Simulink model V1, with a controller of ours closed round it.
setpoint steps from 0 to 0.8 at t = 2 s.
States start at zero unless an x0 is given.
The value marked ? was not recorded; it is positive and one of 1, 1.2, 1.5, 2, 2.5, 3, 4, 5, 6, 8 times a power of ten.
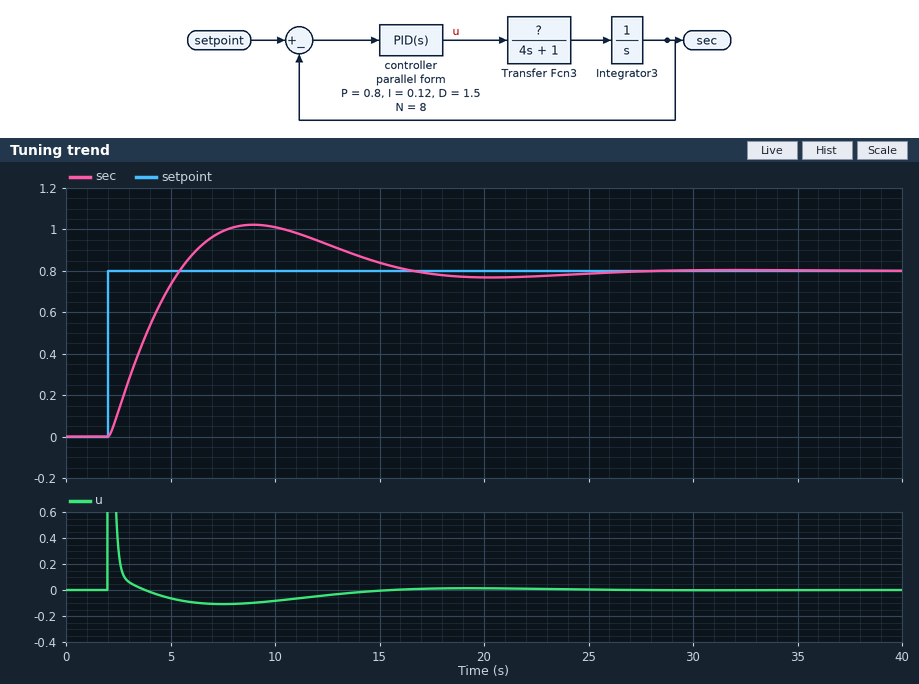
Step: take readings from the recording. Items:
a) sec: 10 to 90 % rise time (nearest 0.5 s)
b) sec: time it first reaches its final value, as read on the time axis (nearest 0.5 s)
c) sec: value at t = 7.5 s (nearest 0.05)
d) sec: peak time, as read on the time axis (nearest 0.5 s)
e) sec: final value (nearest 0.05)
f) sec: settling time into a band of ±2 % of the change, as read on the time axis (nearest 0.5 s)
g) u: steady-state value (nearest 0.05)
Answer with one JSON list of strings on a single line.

["2.5 s", "5.5 s", "1.00", "9.0 s", "0.80", "24.5 s", "0.00"]
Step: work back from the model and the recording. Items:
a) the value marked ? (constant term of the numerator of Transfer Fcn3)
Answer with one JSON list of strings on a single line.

["1"]
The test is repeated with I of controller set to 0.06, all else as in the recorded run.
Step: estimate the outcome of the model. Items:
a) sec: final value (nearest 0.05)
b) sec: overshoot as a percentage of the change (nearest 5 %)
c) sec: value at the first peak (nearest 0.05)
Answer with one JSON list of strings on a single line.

["0.80", "20 %", "0.95"]
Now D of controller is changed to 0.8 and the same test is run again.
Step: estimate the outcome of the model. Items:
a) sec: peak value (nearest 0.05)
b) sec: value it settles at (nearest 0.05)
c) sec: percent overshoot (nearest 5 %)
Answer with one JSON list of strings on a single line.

["1.15", "0.80", "45 %"]
